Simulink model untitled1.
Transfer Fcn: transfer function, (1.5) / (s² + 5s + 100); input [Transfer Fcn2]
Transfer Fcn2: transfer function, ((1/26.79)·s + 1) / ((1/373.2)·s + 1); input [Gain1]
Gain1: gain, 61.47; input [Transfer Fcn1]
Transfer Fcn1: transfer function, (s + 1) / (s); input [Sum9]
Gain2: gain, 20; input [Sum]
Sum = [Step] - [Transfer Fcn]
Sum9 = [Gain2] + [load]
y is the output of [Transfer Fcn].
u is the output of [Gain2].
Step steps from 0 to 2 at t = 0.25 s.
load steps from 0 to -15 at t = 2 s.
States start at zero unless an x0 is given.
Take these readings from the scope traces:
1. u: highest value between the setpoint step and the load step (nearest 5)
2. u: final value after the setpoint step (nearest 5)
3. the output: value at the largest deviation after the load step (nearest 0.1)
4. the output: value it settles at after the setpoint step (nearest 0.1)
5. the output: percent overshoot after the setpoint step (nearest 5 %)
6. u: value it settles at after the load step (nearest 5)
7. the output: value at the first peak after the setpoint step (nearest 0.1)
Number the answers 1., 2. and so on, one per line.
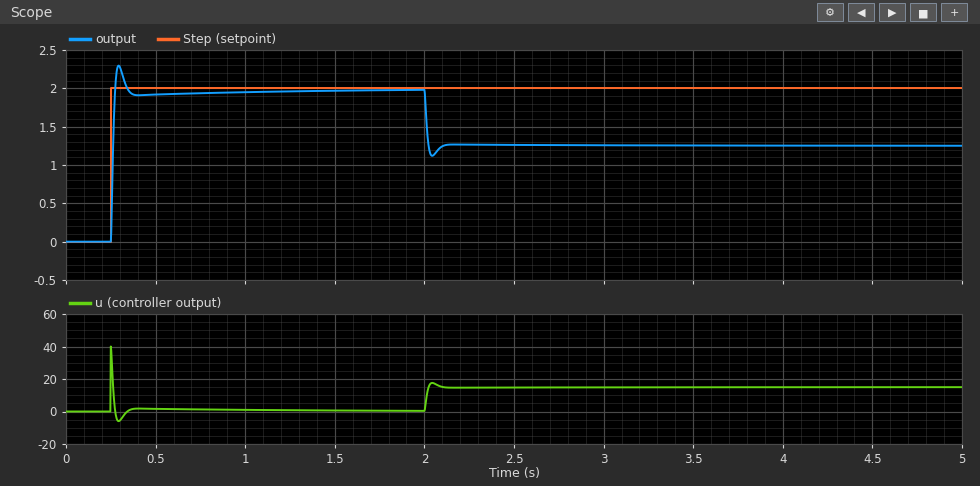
1. 40
2. 0
3. 1.1
4. 2.0
5. 15 %
6. 15
7. 2.3
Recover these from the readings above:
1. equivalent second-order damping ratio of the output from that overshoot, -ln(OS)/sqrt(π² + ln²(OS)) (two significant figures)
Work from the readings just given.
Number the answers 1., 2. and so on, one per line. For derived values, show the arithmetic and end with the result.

1. ln(0.15) = -1.897; 1.897 / sqrt(9.870 + 3.599) = 0.52
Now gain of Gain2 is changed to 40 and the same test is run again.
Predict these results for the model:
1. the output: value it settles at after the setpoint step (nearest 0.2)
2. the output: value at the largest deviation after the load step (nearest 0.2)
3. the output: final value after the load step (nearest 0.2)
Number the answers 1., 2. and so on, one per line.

1. 2.0
2. 1.6
3. 1.6
